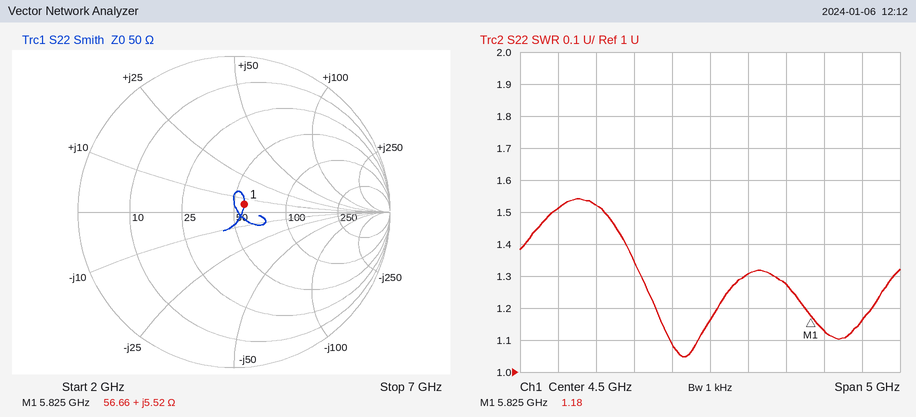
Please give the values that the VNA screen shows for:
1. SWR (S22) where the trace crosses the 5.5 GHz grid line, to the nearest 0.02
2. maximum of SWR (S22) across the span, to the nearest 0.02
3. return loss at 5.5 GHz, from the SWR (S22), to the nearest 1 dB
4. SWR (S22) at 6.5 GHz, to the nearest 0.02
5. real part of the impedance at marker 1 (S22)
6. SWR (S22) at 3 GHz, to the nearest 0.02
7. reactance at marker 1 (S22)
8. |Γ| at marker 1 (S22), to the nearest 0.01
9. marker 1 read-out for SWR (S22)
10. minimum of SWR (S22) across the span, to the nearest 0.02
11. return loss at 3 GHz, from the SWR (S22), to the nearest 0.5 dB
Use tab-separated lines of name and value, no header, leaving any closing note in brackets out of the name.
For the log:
SWR (S22) where the trace crosses the 5.5 GHz grid line, to the nearest 0.02	1.28
maximum of SWR (S22) across the span, to the nearest 0.02	1.54
return loss at 5.5 GHz, from the SWR (S22), to the nearest 1 dB	18 dB
SWR (S22) at 6.5 GHz, to the nearest 0.02	1.16
real part of the impedance at marker 1	56.66 Ω
SWR (S22) at 3 GHz, to the nearest 0.02	1.52
reactance at marker 1	+5.52 Ω
|Γ| at marker 1 (S22), to the nearest 0.01	0.08
marker 1 read-out for SWR	1.18
minimum of SWR (S22) across the span, to the nearest 0.02	1.04
return loss at 3 GHz, from the SWR (S22), to the nearest 0.5 dB	13.5 dB
